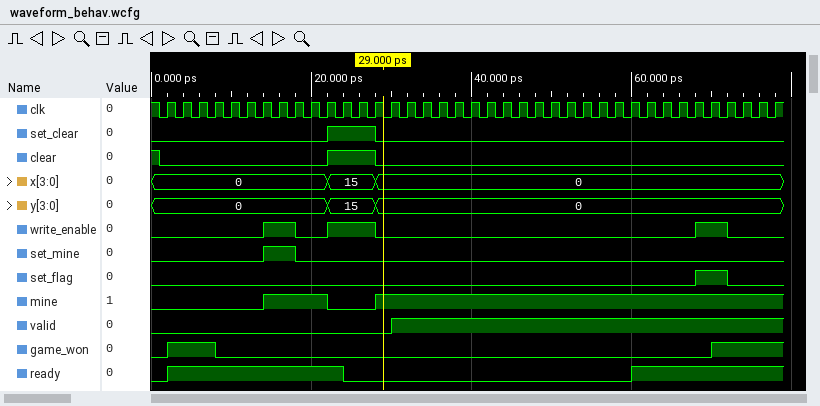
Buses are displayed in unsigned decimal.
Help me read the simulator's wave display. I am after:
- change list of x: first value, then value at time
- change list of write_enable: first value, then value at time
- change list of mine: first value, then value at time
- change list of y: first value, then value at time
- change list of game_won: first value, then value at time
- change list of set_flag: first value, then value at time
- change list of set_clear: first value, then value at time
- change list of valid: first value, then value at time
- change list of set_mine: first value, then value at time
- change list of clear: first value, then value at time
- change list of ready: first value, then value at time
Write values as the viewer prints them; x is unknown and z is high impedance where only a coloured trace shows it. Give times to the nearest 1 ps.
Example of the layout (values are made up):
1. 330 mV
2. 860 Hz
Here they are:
1. 0, 15 at 22 ps, 0 at 28 ps
2. 0, 1 at 14 ps, 0 at 18 ps, 1 at 22 ps, 0 at 28 ps, 1 at 68 ps, 0 at 72 ps
3. 0, 1 at 14 ps, 0 at 22 ps, 1 at 28 ps
4. 0, 15 at 22 ps, 0 at 28 ps
5. 0, 1 at 2 ps, 0 at 8 ps, 1 at 70 ps
6. 0, 1 at 68 ps, 0 at 72 ps
7. 0, 1 at 22 ps, 0 at 28 ps
8. 0, 1 at 30 ps
9. 0, 1 at 14 ps, 0 at 18 ps
10. 1, 0 at 1 ps, 1 at 22 ps, 0 at 28 ps
11. 0, 1 at 2 ps, 0 at 24 ps, 1 at 60 ps
